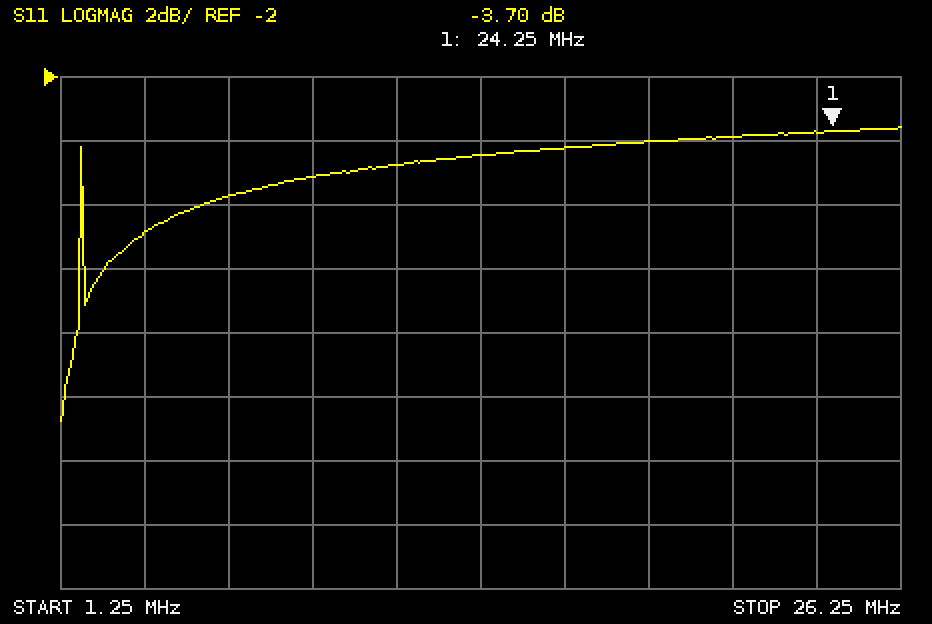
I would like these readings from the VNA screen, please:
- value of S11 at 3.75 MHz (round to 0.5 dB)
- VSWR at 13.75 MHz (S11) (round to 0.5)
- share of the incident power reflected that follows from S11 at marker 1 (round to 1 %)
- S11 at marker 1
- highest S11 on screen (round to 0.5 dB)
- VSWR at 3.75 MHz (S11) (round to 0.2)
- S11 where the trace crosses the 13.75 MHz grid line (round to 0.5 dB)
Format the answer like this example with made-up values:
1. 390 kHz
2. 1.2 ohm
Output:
1. -7.0 dB
2. 4.0
3. 43 %
4. -3.70 dB
5. -3.5 dB
6. 2.6
7. -4.5 dB
